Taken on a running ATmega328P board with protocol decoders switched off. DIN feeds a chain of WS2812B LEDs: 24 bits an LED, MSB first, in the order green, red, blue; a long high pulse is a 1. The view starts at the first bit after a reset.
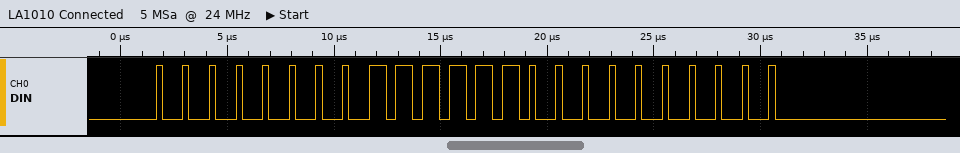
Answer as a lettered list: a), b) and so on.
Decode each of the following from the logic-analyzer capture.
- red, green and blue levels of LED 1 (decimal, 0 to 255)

a) 252, 0, 0
